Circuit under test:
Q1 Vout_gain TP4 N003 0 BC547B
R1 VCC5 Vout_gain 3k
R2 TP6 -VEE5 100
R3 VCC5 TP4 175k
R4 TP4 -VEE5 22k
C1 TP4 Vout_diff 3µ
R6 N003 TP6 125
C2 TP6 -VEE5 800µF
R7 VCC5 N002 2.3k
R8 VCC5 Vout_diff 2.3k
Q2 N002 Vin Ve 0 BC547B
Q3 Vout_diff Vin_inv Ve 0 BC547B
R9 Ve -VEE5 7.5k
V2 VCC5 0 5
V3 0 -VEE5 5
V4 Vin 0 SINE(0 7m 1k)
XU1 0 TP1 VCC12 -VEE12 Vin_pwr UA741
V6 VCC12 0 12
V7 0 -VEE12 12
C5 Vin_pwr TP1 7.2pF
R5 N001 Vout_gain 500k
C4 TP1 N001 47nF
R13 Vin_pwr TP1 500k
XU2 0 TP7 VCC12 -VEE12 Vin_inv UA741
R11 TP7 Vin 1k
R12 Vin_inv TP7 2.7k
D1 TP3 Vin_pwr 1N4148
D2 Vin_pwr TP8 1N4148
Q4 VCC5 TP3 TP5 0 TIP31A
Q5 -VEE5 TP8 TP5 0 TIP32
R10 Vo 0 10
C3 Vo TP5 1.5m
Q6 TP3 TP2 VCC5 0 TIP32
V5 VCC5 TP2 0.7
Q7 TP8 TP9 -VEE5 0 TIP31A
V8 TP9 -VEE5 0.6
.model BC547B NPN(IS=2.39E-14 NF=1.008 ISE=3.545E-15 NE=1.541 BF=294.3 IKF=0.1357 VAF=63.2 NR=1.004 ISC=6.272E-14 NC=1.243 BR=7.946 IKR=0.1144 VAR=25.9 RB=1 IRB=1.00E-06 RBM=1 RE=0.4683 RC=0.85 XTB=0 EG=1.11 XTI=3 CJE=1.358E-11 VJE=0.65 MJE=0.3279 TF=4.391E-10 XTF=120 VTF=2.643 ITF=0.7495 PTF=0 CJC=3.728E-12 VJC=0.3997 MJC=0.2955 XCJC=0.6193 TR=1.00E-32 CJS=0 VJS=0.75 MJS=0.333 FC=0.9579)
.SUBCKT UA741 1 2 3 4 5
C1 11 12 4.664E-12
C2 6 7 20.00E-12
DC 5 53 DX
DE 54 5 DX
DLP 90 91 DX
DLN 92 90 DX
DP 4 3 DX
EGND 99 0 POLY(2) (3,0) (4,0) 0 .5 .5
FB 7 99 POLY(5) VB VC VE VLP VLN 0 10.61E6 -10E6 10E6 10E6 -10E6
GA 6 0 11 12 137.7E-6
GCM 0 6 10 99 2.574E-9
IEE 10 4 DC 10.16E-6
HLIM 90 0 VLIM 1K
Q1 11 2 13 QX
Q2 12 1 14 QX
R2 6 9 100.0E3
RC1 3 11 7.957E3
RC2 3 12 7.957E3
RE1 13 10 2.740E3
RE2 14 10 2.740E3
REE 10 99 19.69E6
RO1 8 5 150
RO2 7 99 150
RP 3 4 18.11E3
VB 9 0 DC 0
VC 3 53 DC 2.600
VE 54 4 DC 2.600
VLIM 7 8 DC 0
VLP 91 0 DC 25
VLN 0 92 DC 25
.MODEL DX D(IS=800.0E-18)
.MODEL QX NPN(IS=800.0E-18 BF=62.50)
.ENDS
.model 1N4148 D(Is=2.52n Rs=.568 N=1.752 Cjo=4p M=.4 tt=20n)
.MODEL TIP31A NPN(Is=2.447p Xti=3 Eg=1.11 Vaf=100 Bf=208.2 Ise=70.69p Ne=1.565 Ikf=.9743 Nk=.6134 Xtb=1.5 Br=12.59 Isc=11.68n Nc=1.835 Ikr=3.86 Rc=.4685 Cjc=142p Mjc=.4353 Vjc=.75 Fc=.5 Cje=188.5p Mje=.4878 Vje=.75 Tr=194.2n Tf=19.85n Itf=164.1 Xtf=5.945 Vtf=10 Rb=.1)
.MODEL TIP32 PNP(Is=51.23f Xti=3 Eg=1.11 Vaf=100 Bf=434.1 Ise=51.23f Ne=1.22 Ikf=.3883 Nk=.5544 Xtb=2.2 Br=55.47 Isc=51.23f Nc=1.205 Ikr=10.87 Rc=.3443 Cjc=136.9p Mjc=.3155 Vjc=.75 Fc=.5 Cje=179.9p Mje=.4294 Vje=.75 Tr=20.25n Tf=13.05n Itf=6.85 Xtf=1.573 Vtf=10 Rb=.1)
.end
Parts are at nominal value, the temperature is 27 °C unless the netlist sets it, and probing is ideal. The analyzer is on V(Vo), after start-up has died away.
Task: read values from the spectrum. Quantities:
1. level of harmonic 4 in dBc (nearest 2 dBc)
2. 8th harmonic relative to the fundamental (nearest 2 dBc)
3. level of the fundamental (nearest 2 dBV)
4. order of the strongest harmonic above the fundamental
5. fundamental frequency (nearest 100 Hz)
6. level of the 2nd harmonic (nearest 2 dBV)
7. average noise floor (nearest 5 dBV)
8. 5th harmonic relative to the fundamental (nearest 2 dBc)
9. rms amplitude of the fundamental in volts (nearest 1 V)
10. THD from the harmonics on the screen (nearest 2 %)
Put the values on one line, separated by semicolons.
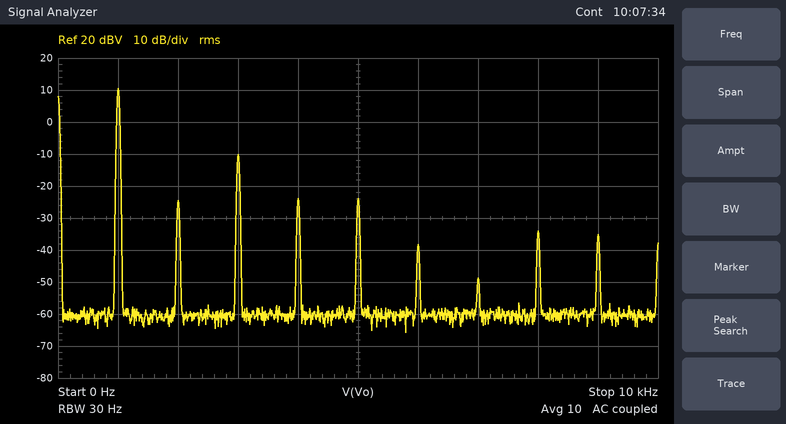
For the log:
-34 dBc; -44 dBc; 10 dBV; 3; 1.0 kHz; -24 dBV; -60 dBV; -34 dBc; 3 V; 10 %
